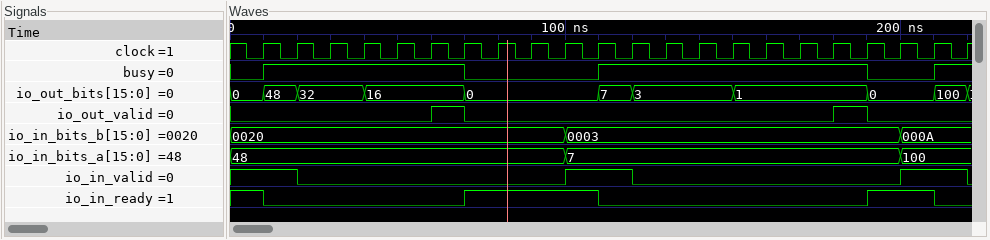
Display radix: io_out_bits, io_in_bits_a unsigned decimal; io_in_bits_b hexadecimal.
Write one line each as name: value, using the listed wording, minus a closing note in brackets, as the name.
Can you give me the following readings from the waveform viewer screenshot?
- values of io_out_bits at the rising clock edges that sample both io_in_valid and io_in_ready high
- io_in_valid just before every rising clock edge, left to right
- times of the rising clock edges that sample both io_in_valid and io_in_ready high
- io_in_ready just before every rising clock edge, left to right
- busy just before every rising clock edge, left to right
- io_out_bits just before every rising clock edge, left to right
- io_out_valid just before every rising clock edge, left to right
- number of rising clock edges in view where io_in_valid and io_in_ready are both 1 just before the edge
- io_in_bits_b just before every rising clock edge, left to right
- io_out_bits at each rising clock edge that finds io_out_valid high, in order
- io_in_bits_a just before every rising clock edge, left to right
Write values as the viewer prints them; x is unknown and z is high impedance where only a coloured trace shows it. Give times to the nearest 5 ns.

values of io_out_bits at the rising clock edges that sample both io_in_valid and io_in_ready high: 0, 0, 0
io_in_valid just before every rising clock edge, left to right: 1 1 0 0 0 0 0 0 0 0 1 1 0 0 0 0 0 0 0 0 1 1
times of the rising clock edges that sample both io_in_valid and io_in_ready high: 10 ns, 110 ns, 210 ns
io_in_ready just before every rising clock edge, left to right: 1 0 0 0 0 0 0 1 1 1 1 0 0 0 0 0 0 0 0 1 1 0
busy just before every rising clock edge, left to right: 0 1 1 1 1 1 1 0 0 0 0 1 1 1 1 1 1 1 1 0 0 1
io_out_bits just before every rising clock edge, left to right: 0, 48, 32, 32, 16, 16, 16, 0, 0, 0, 0, 7, 3, 3, 3, 1, 1, 1, 1, 0, 0, 100
io_out_valid just before every rising clock edge, left to right: 0 0 0 0 0 0 1 0 0 0 0 0 0 0 0 0 0 0 1 0 0 0
number of rising clock edges in view where io_in_valid and io_in_ready are both 1 just before the edge: 3
io_in_bits_b just before every rising clock edge, left to right: 0020, 0020, 0020, 0020, 0020, 0020, 0020, 0020, 0020, 0020, 0003, 0003, 0003, 0003, 0003, 0003, 0003, 0003, 0003, 0003, 000A, 000A
io_out_bits at each rising clock edge that finds io_out_valid high, in order: 16, 1
io_in_bits_a just before every rising clock edge, left to right: 48, 48, 48, 48, 48, 48, 48, 48, 48, 48, 7, 7, 7, 7, 7, 7, 7, 7, 7, 7, 100, 100
